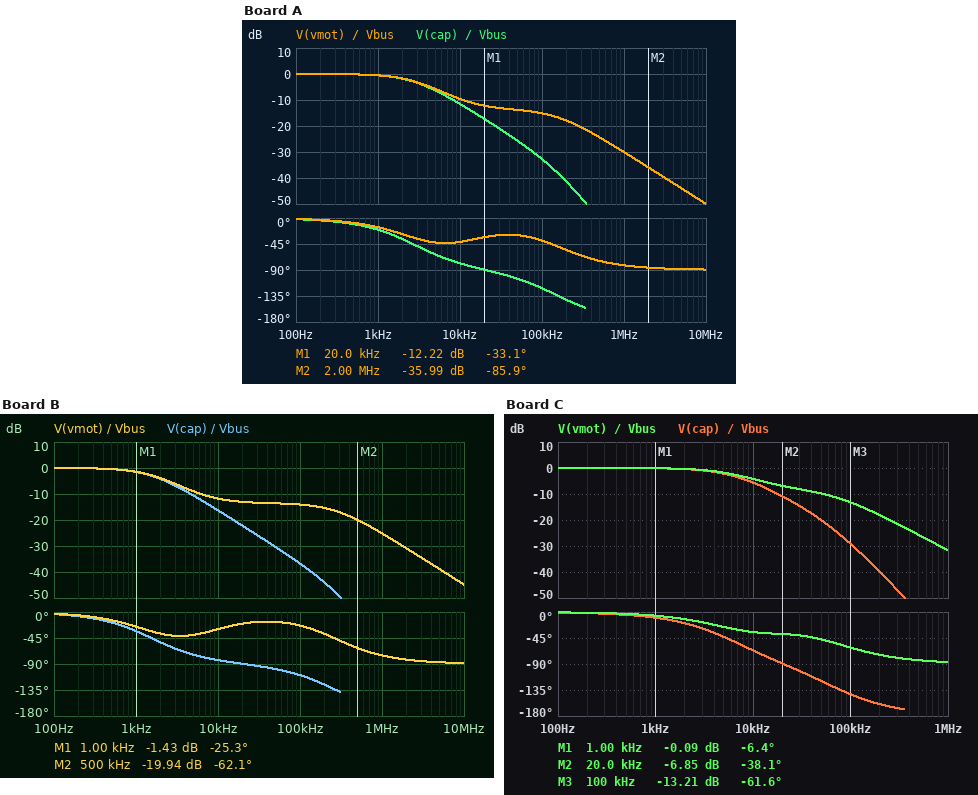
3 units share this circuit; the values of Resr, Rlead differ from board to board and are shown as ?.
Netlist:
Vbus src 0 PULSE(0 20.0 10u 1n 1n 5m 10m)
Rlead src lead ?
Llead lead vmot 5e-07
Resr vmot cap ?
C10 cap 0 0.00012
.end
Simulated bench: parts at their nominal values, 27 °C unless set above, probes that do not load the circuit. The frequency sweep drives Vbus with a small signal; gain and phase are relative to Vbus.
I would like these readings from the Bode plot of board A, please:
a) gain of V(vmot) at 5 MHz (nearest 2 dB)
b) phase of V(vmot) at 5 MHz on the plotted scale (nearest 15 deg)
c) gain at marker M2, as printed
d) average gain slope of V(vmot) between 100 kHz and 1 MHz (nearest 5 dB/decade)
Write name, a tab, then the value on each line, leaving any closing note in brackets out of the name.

gain of V(vmot) at 5 MHz	-44 dB
phase of V(vmot) at 5 MHz on the plotted scale	-90 deg
gain at marker M2, as printed	-35.99 dB
average gain slope of V(vmot) between 100 kHz and 1 MHz	-15 dB/decade
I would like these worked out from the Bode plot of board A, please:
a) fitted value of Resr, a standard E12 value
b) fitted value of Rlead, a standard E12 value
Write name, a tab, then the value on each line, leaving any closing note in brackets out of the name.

fitted value of Resr, a standard E12 value	0.1 Ω
fitted value of Rlead, a standard E12 value	0.39 Ω
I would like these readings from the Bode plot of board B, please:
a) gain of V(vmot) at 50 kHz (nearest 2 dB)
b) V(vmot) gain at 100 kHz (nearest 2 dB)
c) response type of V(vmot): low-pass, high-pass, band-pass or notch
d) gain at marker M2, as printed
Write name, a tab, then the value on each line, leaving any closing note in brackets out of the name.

gain of V(vmot) at 50 kHz	-14 dB
V(vmot) gain at 100 kHz	-14 dB
response type of V(vmot): low-pass, high-pass, band-pass or notch	low-pass
gain at marker M2, as printed	-19.94 dB
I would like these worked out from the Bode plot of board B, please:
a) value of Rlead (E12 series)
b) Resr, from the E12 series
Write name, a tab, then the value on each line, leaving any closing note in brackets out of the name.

value of Rlead	0.68 Ω
Resr, from the E12 series	0.18 Ω
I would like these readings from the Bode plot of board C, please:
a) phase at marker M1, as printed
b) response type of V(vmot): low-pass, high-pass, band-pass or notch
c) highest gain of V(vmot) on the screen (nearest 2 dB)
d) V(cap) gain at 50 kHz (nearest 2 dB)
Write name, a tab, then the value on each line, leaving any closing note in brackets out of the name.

phase at marker M1, as printed	-6.4 deg
response type of V(vmot): low-pass, high-pass, band-pass or notch	low-pass
highest gain of V(vmot) on the screen	0 dB
V(cap) gain at 50 kHz	-20 dB
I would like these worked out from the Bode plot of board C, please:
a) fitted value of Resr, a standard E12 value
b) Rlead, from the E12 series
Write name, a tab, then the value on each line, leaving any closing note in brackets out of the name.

fitted value of Resr, a standard E12 value	0.082 Ω
Rlead, from the E12 series	0.15 Ω
